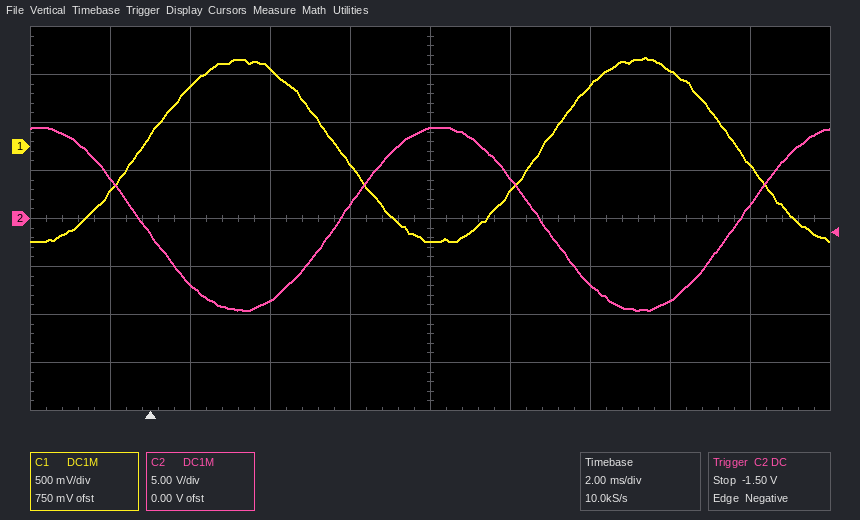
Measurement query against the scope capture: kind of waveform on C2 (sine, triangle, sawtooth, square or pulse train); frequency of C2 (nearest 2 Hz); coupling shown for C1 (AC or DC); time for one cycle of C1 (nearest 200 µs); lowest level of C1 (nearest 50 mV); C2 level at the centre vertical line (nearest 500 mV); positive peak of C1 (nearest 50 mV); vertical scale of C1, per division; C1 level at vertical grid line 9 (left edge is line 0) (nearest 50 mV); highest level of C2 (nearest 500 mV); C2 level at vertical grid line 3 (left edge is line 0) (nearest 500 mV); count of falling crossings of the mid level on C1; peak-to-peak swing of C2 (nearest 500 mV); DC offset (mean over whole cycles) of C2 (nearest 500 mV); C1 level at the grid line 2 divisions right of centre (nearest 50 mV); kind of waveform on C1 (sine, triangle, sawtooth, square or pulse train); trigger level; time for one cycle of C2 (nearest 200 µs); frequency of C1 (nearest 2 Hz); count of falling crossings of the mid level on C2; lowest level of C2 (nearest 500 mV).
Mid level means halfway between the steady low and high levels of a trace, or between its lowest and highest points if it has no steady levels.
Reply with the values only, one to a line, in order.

sine
100 Hz
DC
10.0 ms
-1.00 V
9.5 V
950 mV
500 mV
-200 mV
9.5 V
-8.5 V
2
19.0 V
0.0 V
650 mV
sine
-1.50 V
10.0 ms
100 Hz
2
-9.5 V
